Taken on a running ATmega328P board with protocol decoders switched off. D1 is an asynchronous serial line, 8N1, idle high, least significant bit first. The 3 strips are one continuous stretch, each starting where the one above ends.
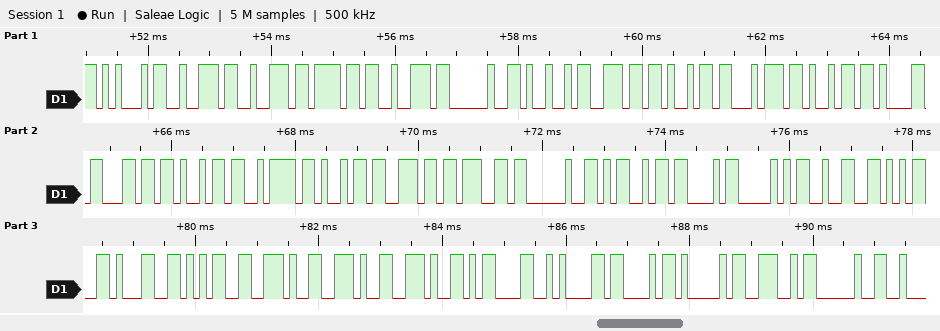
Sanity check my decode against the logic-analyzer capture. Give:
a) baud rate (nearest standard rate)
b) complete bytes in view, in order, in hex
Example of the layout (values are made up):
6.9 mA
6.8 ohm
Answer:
9600 baud
45 72 72 6F 72 20 49 6E 69 74 69 61 6C 69 7A 69 6E 67 20 4D 43 50 32 35 31 35 2E 2E 2E 0D 0A 43 41 4E 20
